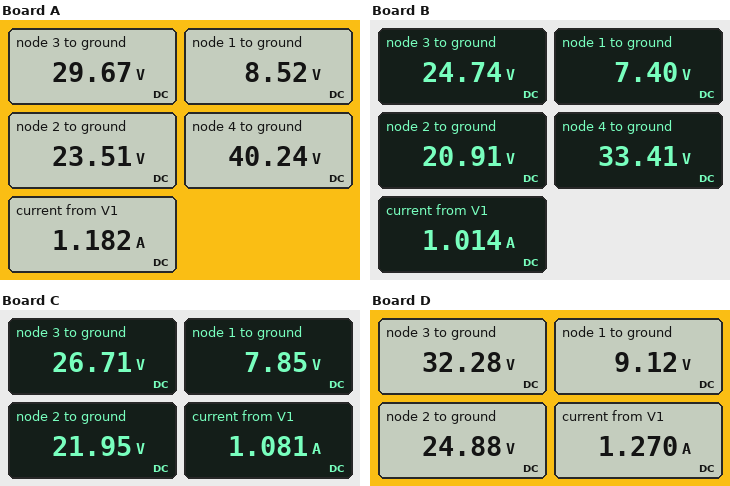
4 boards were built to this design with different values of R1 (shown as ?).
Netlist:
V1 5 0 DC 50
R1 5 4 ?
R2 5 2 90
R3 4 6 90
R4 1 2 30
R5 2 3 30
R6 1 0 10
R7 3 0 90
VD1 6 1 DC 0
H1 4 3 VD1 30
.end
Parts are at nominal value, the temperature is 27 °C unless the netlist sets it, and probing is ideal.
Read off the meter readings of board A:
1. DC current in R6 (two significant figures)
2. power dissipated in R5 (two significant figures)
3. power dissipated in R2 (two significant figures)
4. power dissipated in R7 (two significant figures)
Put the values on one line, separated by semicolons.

850 mA; 1.3 W; 7.8 W; 9.8 W
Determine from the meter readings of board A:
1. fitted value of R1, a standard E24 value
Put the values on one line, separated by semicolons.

11 Ω
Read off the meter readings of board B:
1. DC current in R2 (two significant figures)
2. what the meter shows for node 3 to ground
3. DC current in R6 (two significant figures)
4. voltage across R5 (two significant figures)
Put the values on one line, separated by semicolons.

320 mA; 24.74 V; 740 mA; 3.8 V
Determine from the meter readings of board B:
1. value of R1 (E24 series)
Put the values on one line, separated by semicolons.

24 Ω
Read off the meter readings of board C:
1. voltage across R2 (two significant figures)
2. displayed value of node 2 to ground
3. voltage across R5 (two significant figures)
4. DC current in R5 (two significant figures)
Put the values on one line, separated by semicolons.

28 V; 21.95 V; 4.8 V; 160 mA
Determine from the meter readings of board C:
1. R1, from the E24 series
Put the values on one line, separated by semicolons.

18 Ω
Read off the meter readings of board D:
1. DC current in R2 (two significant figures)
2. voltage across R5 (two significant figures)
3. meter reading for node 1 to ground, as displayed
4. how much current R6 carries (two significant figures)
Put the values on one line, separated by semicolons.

280 mA; 7.4 V; 9.12 V; 910 mA
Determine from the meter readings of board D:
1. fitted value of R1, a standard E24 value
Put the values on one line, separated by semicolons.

6.2 Ω
